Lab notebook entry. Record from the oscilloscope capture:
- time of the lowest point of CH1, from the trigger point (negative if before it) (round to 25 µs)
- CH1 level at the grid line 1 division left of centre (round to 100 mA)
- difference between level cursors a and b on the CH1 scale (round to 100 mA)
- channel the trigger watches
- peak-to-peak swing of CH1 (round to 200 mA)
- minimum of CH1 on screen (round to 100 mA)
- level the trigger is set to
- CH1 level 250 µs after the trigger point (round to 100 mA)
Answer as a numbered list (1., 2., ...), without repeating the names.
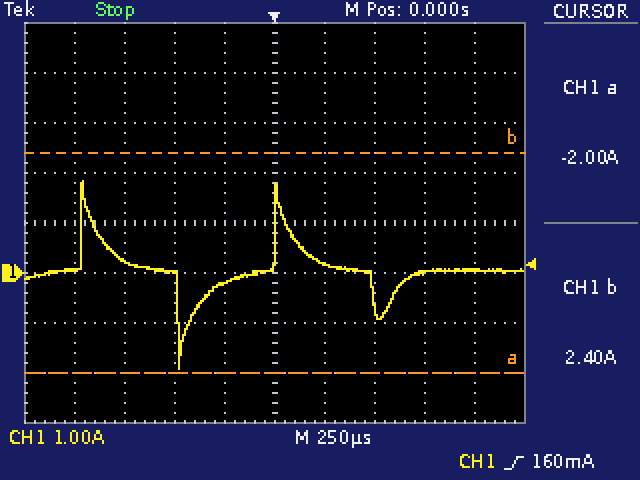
1. -475 µs
2. -200 mA
3. 4.4 A
4. CH1
5. 3.8 A
6. -1.9 A
7. 160 mA
8. 200 mA
